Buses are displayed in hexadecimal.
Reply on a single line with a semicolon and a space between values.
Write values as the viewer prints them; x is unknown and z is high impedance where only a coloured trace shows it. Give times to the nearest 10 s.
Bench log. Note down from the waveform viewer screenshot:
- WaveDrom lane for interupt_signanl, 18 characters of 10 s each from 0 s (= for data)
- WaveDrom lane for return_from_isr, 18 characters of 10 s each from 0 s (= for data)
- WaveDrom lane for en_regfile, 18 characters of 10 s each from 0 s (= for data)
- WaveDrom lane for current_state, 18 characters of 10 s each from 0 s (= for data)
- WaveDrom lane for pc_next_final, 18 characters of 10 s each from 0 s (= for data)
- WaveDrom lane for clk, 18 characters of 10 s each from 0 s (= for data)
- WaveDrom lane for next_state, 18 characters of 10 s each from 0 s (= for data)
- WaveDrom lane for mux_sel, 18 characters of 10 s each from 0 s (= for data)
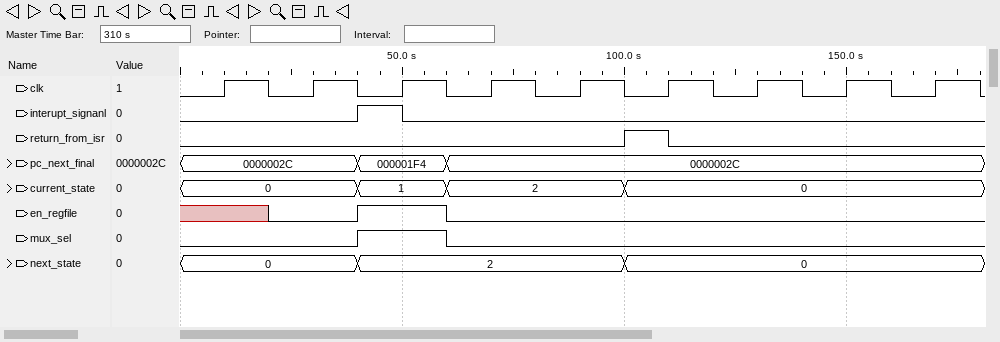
{name: 'interupt_signanl', wave: '0...10............'}; {name: 'return_from_isr', wave: '0.........10......'}; {name: 'en_regfile', wave: 'x.0.1.0...........'}; {name: 'current_state', wave: '=...=.=...=.......', data: '0 1 2 0'}; {name: 'pc_next_final', wave: '=...=.=...........', data: '0000002C 000001F4 0000002C'}; {name: 'clk', wave: '010101010101010101'}; {name: 'next_state', wave: '=...=.....=.......', data: '0 2 0'}; {name: 'mux_sel', wave: '0...1.0...........'}
